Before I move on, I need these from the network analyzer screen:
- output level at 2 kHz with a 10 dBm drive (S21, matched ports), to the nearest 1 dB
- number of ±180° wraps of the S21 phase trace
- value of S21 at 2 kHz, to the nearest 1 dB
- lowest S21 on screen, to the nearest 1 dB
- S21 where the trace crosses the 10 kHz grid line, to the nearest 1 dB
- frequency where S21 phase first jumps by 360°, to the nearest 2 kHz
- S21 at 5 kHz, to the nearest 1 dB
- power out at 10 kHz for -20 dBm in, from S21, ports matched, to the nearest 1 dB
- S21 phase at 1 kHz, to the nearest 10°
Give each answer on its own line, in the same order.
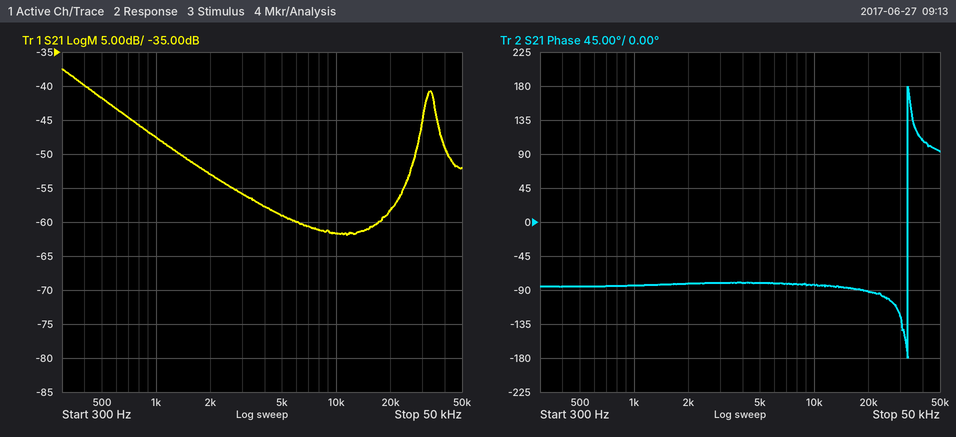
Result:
-43 dBm
1
-53 dB
-62 dB
-62 dB
34 kHz
-59 dB
-82 dBm
-80°
